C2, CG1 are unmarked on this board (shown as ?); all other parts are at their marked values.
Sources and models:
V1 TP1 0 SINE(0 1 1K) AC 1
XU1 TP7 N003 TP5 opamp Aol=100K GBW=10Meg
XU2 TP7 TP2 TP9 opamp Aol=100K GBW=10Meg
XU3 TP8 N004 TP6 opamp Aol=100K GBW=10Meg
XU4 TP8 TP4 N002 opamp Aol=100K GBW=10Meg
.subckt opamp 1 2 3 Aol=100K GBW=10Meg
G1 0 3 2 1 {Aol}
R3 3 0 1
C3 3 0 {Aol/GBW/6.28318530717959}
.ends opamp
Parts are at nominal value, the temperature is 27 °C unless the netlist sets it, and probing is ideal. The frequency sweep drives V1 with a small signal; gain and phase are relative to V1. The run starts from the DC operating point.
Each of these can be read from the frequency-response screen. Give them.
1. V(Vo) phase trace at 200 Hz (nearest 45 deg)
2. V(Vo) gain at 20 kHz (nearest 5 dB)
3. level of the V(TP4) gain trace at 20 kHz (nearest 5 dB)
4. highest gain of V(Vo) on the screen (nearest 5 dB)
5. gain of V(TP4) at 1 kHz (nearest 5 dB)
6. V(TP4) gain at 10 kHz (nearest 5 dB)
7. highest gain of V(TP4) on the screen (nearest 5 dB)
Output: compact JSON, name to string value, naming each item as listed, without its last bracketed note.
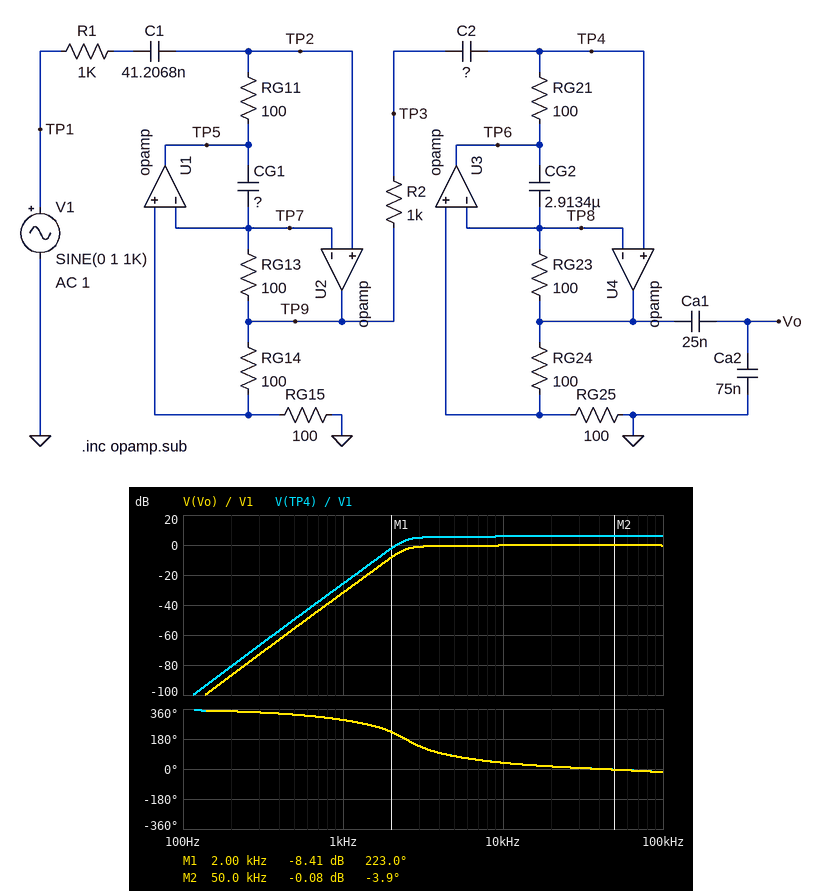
{"V(Vo) phase trace at 200 Hz": "360 deg", "V(Vo) gain at 20 kHz": "0 dB", "level of the V(TP4) gain trace at 20 kHz": "5 dB", "highest gain of V(Vo) on the screen": "0 dB", "gain of V(TP4) at 1 kHz": "-25 dB", "V(TP4) gain at 10 kHz": "5 dB", "highest gain of V(TP4) on the screen": "5 dB"}
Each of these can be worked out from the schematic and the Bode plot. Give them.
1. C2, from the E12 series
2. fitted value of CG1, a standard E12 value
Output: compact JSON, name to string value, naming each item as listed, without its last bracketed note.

{"C2, from the E12 series": "150 nF", "fitted value of CG1, a standard E12 value": "10 µF"}
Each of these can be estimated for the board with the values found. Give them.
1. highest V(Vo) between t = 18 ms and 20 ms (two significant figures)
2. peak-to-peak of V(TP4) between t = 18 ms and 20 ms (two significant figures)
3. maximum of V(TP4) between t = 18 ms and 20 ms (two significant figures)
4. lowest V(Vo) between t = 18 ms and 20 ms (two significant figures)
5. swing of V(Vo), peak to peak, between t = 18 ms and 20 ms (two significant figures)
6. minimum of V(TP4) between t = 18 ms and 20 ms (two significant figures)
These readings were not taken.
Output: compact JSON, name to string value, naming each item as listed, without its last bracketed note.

{"highest V(Vo) between t = 18 ms and 20 ms": "26 mV", "peak-to-peak of V(TP4) between t = 18 ms and 20 ms": "100 mV", "maximum of V(TP4) between t = 18 ms and 20 ms": "51 mV", "lowest V(Vo) between t = 18 ms and 20 ms": "-26 mV", "swing of V(Vo), peak to peak, between t = 18 ms and 20 ms": "51 mV", "minimum of V(TP4) between t = 18 ms and 20 ms": "-51 mV"}
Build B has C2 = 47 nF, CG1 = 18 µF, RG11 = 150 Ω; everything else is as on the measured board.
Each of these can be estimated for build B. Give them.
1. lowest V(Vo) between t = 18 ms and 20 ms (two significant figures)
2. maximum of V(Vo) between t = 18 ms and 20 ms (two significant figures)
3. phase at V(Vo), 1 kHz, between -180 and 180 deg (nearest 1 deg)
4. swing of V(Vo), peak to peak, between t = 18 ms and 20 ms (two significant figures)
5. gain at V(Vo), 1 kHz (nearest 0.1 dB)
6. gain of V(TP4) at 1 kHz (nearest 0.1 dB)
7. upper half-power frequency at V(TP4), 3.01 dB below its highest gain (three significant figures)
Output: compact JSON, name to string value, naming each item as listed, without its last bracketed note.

{"lowest V(Vo) between t = 18 ms and 20 ms": "-39 mV", "maximum of V(Vo) between t = 18 ms and 20 ms": "39 mV", "phase at V(Vo), 1 kHz, between -180 and 180 deg": "-42 deg", "swing of V(Vo), peak to peak, between t = 18 ms and 20 ms": "78 mV", "gain at V(Vo), 1 kHz": "-28.2 dB", "gain of V(TP4) at 1 kHz": "-22.2 dB", "upper half-power frequency at V(TP4), 3.01 dB below its highest gain": "330 kHz"}
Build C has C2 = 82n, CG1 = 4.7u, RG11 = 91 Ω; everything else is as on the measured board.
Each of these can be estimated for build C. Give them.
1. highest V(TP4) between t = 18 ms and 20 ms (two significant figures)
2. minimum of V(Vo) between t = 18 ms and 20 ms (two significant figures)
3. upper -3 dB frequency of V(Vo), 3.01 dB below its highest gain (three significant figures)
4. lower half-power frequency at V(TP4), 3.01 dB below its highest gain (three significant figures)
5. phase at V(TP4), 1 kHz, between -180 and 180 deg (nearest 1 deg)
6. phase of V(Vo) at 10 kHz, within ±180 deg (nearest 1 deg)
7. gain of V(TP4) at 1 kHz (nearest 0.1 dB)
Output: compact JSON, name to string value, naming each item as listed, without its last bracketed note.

{"highest V(TP4) between t = 18 ms and 20 ms": "13 mV", "minimum of V(Vo) between t = 18 ms and 20 ms": "-6.5 mV", "upper -3 dB frequency of V(Vo), 3.01 dB below its highest gain": "279 kHz", "lower half-power frequency at V(TP4), 3.01 dB below its highest gain": "3.87 kHz", "phase at V(TP4), 1 kHz, between -180 and 180 deg": "-45 deg", "phase of V(Vo) at 10 kHz, within ±180 deg": "52 deg", "gain of V(TP4) at 1 kHz": "-37.7 dB"}
